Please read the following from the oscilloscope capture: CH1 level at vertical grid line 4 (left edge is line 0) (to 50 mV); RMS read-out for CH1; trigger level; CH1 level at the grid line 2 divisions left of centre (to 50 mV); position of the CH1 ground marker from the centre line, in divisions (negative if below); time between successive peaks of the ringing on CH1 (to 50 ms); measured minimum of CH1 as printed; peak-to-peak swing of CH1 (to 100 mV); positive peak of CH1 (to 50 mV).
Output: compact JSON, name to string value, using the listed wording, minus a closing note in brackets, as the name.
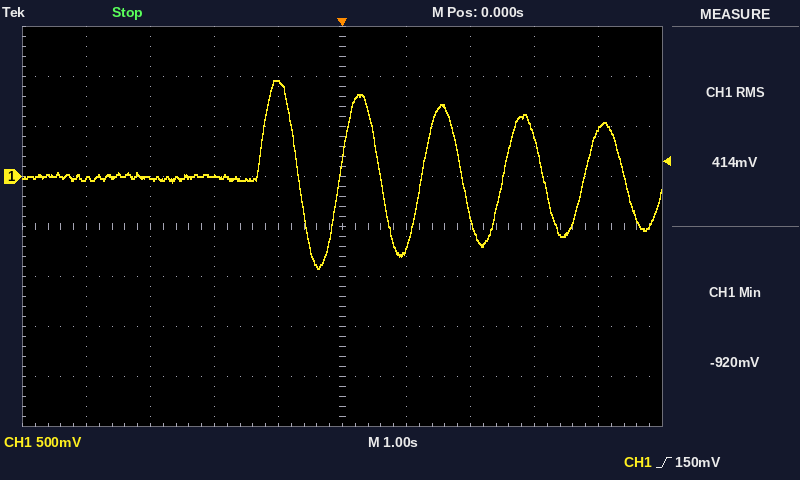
{"CH1 level at vertical grid line 4 (left edge is line 0)": "950 mV", "RMS read-out for CH1": "414 mV", "trigger level": "150 mV", "CH1 level at the grid line 2 divisions left of centre": "0 mV", "position of the CH1 ground marker from the centre line, in divisions": "+1.0 div", "time between successive peaks of the ringing on CH1": "1.30 s", "measured minimum of CH1 as printed": "-920 mV", "peak-to-peak swing of CH1": "1.90 V", "positive peak of CH1": "950 mV"}
